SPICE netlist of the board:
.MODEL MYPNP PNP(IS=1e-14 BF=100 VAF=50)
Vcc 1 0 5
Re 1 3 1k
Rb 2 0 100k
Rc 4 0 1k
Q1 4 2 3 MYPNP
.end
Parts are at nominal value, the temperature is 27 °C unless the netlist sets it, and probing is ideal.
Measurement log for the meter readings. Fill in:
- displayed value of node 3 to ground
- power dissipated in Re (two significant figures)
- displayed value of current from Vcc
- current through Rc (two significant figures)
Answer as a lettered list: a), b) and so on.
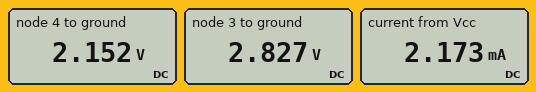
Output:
a) 2.827 V
b) 4.7 mW
c) 2.173 mA
d) 2.2 mA
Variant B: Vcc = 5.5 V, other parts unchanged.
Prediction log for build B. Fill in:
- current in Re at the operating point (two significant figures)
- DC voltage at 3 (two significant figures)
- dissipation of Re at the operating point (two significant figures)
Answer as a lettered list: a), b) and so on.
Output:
a) 2.4 mA
b) 3.1 V
c) 5.9 mW
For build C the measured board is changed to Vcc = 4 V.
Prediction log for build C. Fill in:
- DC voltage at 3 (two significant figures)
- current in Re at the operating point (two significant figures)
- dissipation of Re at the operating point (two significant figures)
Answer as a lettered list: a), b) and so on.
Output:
a) 2.3 V
b) 1.7 mA
c) 2.8 mW
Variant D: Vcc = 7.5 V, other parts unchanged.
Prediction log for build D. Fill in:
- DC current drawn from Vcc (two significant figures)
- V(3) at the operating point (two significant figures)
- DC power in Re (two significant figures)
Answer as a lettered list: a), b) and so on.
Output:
a) 3.4 mA
b) 4.1 V
c) 12 mW
